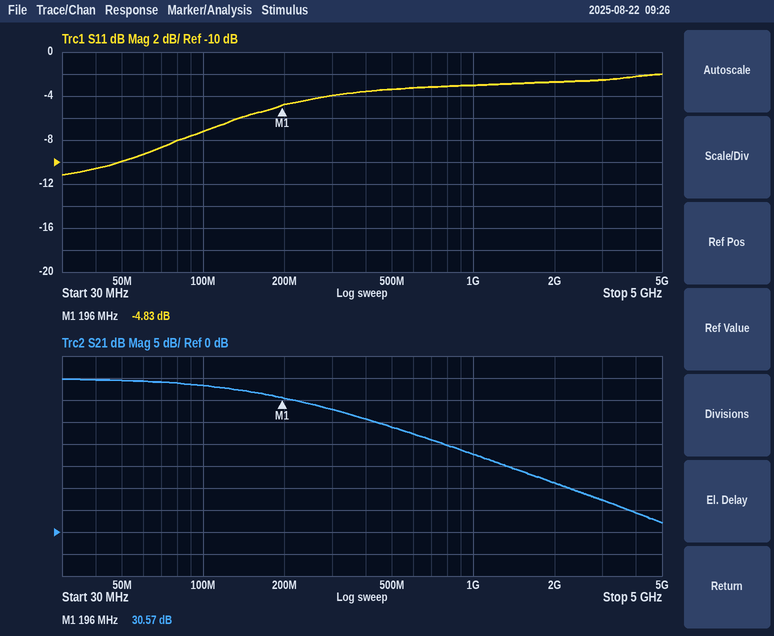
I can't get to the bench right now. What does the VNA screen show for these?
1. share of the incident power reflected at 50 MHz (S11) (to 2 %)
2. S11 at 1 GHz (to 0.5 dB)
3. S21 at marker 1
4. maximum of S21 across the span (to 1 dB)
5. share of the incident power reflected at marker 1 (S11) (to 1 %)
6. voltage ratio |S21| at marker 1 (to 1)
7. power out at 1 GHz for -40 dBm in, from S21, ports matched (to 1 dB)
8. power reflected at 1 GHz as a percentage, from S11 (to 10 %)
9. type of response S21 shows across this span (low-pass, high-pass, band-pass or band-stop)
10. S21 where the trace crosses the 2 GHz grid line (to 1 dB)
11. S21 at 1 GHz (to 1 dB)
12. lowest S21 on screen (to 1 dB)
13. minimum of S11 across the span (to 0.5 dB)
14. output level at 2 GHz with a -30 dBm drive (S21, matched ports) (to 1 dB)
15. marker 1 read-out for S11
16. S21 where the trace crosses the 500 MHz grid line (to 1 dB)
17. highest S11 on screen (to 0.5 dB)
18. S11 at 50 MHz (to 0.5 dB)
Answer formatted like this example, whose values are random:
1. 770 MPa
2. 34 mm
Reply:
1. 10 %
2. -3.0 dB
3. 30.57 dB
4. 35 dB
5. 33 %
6. 34
7. -22 dBm
8. 50 %
9. low-pass
10. 11 dB
11. 18 dB
12. 2 dB
13. -11.0 dB
14. -19 dBm
15. -4.83 dB
16. 24 dB
17. -2.0 dB
18. -10.0 dB
